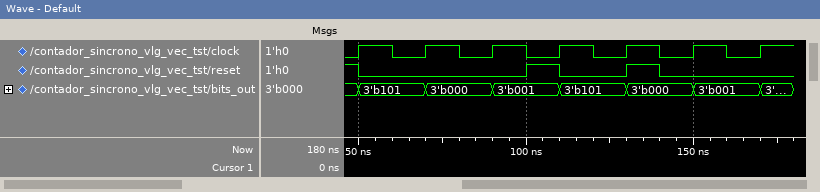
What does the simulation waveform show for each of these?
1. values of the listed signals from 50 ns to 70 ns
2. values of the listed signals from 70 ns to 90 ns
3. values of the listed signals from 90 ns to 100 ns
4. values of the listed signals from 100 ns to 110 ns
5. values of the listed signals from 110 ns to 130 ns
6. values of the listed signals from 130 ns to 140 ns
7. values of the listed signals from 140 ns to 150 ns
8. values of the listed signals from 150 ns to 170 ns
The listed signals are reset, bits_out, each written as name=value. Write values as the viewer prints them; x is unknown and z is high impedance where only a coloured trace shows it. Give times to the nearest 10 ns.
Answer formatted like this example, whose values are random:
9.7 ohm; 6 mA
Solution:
reset=0, bits_out=3'b101; reset=0, bits_out=3'b000; reset=0, bits_out=3'b001; reset=1, bits_out=3'b001; reset=0, bits_out=3'b101; reset=1, bits_out=3'b000; reset=0, bits_out=3'b000; reset=0, bits_out=3'b001
